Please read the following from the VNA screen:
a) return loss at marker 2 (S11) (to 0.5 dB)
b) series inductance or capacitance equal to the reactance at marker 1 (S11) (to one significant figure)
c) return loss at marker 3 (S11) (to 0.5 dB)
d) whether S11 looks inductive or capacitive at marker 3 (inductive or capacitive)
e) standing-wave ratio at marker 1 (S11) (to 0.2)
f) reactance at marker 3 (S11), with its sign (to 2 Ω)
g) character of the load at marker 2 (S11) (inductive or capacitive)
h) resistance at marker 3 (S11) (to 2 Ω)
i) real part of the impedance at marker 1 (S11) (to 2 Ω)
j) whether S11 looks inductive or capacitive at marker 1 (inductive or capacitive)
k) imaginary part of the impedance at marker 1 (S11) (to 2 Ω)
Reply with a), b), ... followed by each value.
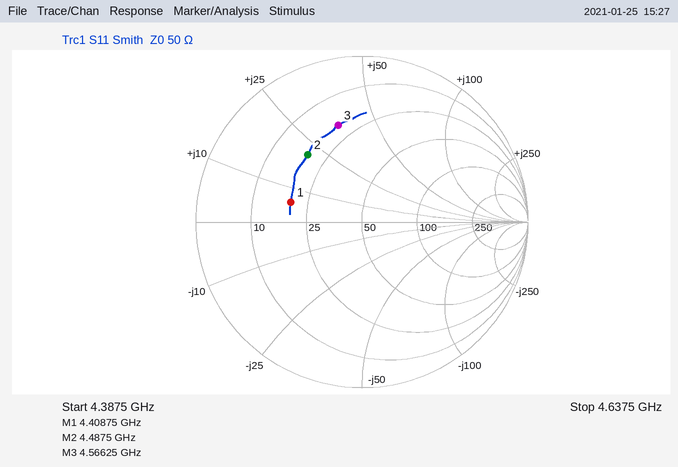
a) 5.5 dB
b) 200 pH
c) 4.5 dB
d) inductive
e) 2.6
f) +36 Ω
g) inductive
h) 20 Ω
i) 20 Ω
j) inductive
k) +6 Ω
